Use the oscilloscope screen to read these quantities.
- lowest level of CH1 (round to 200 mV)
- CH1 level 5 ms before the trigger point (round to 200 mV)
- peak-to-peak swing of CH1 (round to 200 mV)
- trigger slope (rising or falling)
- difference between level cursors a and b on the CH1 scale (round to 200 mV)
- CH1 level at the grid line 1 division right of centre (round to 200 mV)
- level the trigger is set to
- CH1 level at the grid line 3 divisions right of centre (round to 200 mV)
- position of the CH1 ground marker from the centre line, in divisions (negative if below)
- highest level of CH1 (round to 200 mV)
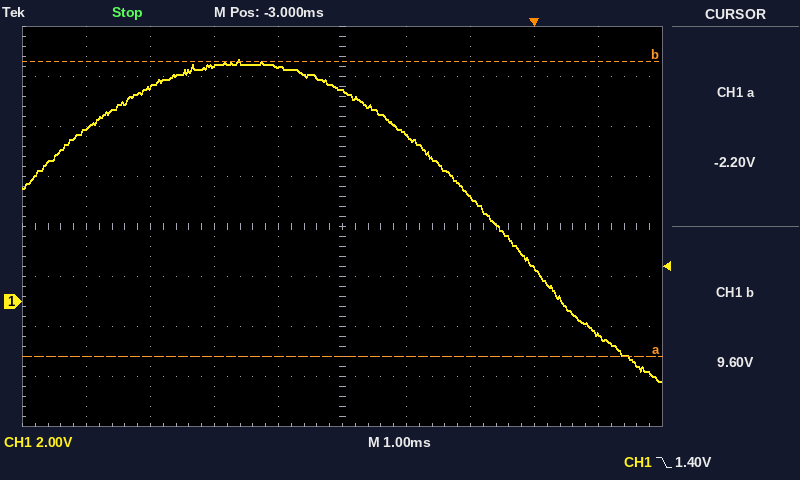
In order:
-3.2 V
9.4 V
12.8 V
falling
11.8 V
6.6 V
1.40 V
1.4 V
-1.5 div
9.6 V
